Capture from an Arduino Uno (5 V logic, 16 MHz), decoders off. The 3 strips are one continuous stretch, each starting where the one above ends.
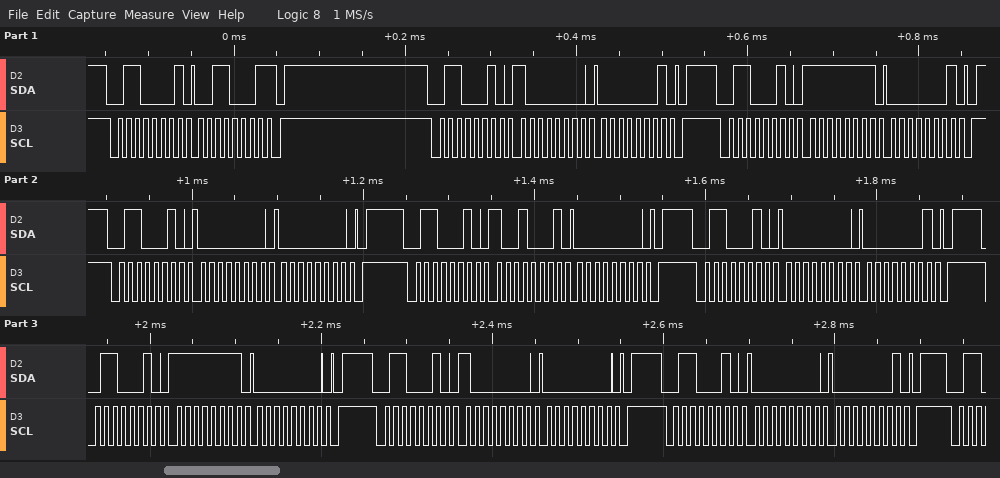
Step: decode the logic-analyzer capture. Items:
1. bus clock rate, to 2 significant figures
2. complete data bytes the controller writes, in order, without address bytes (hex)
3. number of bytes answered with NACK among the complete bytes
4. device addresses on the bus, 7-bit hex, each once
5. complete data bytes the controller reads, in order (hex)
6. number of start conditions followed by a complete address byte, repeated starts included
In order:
100 kHz
80 01 FF 01 00 00 91 00 00 01 FF 00 80 00 00 01
1
0x30 0x31
31
9
